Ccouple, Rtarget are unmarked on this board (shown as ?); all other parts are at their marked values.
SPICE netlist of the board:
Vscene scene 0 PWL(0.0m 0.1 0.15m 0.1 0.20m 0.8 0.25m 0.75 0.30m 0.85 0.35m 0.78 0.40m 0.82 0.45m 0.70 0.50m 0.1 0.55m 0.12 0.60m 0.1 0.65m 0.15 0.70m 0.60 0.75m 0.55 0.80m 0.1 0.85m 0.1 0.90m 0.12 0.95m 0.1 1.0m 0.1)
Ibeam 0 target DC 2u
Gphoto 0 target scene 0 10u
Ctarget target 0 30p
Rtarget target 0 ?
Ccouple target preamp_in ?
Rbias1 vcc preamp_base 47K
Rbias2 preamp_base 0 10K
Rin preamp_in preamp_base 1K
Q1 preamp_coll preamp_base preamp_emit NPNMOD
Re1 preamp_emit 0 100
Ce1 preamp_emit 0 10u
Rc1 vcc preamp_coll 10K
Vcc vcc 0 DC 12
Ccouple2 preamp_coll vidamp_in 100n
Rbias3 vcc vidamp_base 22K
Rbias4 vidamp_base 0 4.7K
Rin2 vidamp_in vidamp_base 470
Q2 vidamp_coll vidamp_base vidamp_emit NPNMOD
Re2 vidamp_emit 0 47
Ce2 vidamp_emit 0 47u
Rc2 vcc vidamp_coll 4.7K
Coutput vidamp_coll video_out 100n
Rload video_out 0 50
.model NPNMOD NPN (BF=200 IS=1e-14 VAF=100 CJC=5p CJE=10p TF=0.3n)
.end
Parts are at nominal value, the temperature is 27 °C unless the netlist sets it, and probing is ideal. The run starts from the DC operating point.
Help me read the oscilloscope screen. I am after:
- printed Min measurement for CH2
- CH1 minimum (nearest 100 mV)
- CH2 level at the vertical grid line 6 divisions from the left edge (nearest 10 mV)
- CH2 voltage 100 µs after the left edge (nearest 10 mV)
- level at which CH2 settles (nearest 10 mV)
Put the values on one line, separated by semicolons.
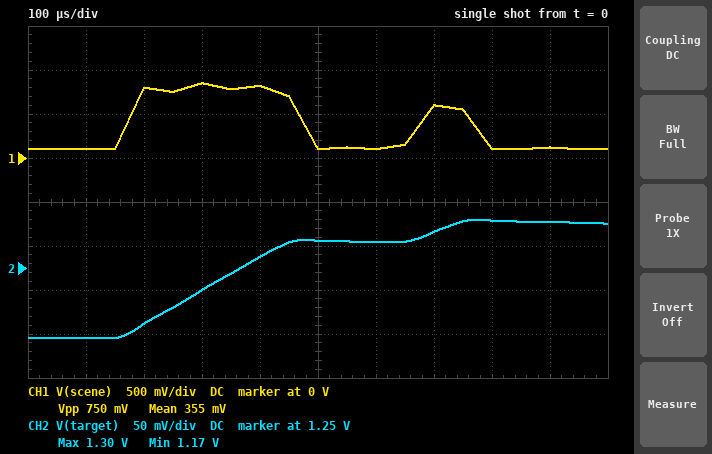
1.17 V; 100 mV; 1.28 V; 1.17 V; 1.30 V
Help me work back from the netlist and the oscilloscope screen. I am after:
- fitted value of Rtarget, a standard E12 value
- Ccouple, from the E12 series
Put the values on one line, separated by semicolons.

390 kΩ; 18 nF
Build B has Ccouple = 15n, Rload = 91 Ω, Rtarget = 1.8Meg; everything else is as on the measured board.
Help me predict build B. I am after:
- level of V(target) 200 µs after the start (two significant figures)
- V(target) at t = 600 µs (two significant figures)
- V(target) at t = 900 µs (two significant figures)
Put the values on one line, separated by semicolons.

5.4 V; 5.5 V; 5.6 V
